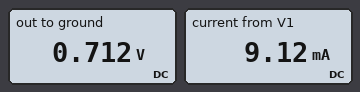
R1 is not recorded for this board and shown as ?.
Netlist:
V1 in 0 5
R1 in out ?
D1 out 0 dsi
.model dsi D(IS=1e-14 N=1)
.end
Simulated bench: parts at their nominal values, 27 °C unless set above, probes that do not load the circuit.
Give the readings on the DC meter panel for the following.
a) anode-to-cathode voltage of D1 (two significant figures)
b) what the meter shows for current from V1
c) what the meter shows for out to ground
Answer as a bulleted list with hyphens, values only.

- 710 mV
- 9.12 mA
- 0.712 V
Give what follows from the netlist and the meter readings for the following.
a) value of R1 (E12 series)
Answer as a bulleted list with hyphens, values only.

- 470 Ω
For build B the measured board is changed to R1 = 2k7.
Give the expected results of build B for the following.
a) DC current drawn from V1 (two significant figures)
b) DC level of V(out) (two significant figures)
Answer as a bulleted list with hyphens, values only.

- 1.6 mA
- 670 mV
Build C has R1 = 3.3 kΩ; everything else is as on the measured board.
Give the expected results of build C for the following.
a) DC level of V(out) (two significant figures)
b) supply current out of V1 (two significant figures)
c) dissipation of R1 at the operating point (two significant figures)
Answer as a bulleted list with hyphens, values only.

- 660 mV
- 1.3 mA
- 5.7 mW
